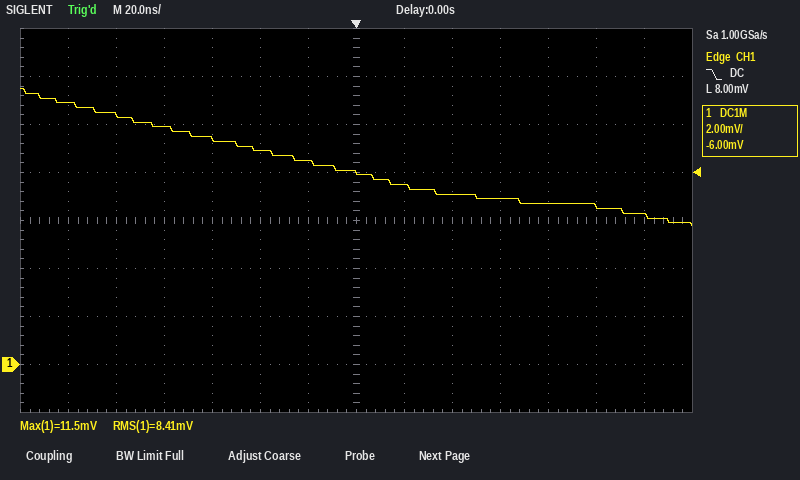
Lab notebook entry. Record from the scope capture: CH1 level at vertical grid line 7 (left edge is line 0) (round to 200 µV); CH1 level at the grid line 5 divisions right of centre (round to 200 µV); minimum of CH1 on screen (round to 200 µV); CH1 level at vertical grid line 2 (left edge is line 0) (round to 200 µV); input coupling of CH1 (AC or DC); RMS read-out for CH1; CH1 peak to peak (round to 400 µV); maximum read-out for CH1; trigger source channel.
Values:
8.0 mV
6.6 mV
5.8 mV
10.4 mV
DC
8.41 mV
5.6 mV
11.5 mV
CH1
